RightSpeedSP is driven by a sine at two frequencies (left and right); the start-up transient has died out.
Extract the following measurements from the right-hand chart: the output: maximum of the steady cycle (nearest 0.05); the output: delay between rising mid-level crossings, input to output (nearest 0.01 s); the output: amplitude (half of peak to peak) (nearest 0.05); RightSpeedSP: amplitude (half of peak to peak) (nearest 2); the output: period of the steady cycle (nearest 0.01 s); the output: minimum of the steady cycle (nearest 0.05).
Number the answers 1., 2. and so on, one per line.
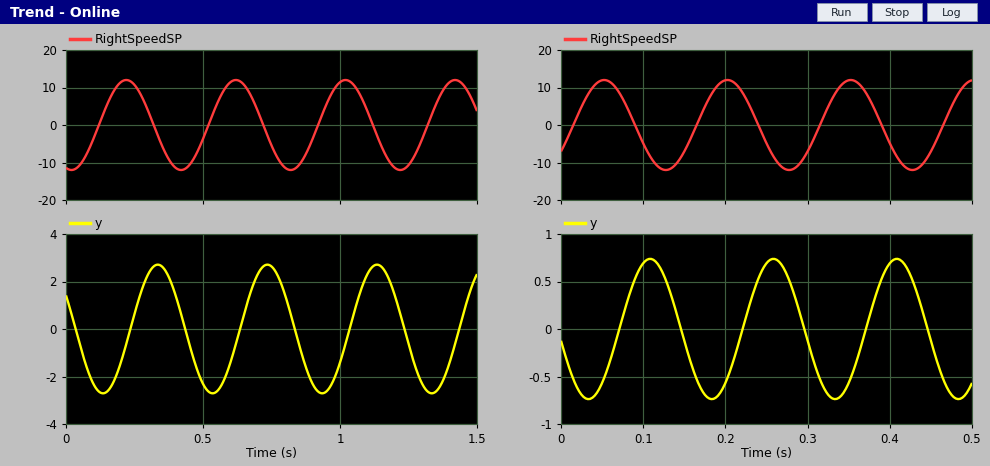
1. 0.75
2. 0.06 s
3. 0.75
4. 12
5. 0.15 s
6. -0.75
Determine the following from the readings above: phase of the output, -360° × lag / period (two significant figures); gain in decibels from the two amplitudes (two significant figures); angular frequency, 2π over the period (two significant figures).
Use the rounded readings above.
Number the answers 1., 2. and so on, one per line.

1. -140°
2. -24 dB
3. 42 rad/s
